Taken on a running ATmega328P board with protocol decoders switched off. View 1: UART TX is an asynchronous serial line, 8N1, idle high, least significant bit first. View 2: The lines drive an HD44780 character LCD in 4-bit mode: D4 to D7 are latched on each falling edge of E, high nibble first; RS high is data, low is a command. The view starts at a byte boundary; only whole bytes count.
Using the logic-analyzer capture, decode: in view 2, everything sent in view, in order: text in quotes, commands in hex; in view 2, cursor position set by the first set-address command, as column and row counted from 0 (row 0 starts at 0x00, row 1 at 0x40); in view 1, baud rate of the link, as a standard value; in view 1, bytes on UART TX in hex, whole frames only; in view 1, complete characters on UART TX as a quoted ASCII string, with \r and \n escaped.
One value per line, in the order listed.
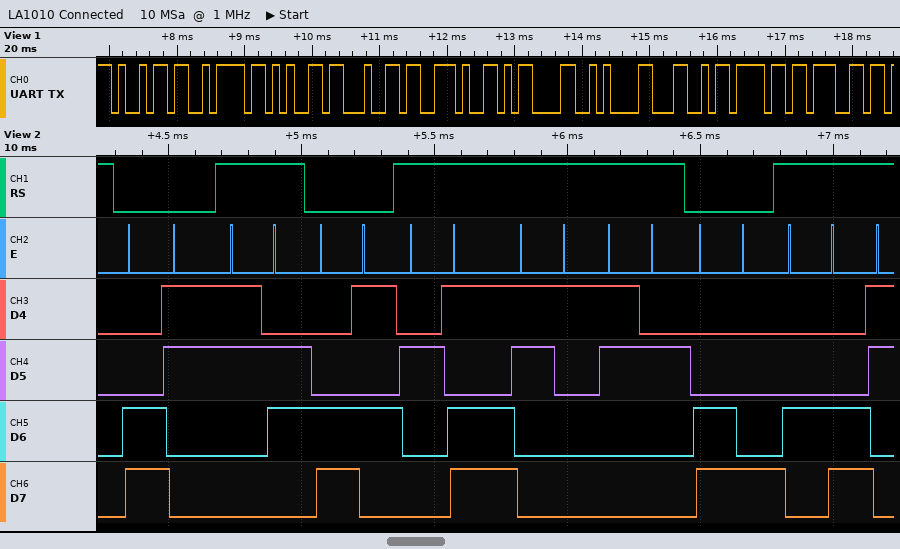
0xC3 "6" 0xC5 "-12" 0xC8 "L"
column 3, row 1
9600 baud
69 7A 65 64 2E 0D 0A 4C 6F 67
"ized.\r\nLog"
